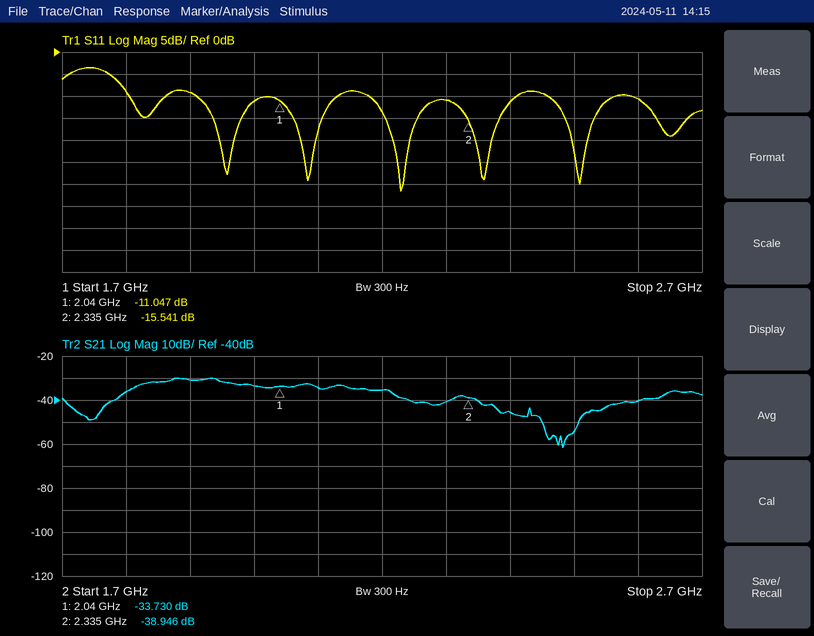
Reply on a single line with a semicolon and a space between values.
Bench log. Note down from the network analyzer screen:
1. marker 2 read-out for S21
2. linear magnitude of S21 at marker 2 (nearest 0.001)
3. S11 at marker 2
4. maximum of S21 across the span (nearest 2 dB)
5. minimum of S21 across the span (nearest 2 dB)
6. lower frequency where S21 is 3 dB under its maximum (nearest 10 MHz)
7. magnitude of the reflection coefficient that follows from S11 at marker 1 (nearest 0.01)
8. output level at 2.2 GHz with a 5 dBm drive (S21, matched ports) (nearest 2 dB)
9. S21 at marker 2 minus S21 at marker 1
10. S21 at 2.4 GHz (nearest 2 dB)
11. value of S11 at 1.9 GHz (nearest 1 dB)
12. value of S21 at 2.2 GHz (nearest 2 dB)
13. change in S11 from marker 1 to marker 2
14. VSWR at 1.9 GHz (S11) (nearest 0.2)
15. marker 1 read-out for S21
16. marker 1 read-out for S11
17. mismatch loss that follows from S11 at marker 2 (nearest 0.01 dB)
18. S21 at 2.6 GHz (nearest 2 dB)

-38.946 dB; 0.011; -15.541 dB; -30 dB; -62 dB; 1.82 GHz; 0.28; -30 dBm; -5.216 dB; -46 dB; -9 dB; -36 dB; -4.494 dB; 2.0; -33.730 dB; -11.047 dB; 0.12 dB; -40 dB
